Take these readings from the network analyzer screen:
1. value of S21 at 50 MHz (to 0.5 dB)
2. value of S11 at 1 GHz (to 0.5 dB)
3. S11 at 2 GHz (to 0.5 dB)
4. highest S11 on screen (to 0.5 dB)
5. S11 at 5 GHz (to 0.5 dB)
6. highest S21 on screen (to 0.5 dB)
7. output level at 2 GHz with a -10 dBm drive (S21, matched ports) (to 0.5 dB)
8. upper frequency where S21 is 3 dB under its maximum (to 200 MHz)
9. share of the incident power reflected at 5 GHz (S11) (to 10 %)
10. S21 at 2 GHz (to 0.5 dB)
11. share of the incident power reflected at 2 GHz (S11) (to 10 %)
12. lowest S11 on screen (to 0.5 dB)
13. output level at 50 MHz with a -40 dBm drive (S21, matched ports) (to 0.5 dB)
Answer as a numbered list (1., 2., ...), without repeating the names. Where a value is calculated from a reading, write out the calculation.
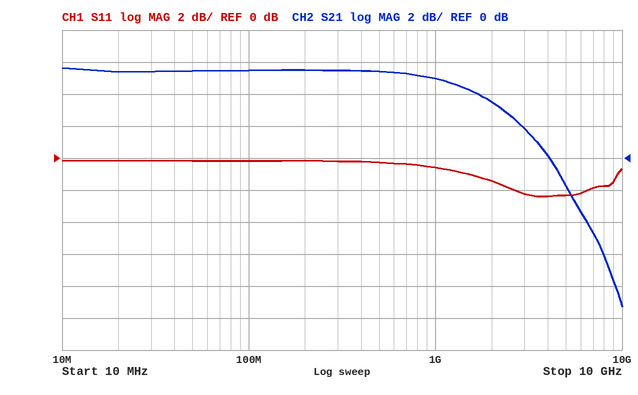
1. 5.5 dB
2. -0.5 dB
3. -1.5 dB
4. 0.0 dB
5. -2.5 dB
6. 5.5 dB
7. -10 dBm + (3.5 dB) = -6.5 dBm
8. 2.6 GHz
9. 10^(-2.5/10) ≈ 56.2 %, so 60 % to the nearest 10 %
10. 3.5 dB
11. 10^(-1.5/10) ≈ 70.8 %, so 70 % to the nearest 10 %
12. -2.5 dB
13. -40 dBm + (5.5 dB) = -34.5 dBm
